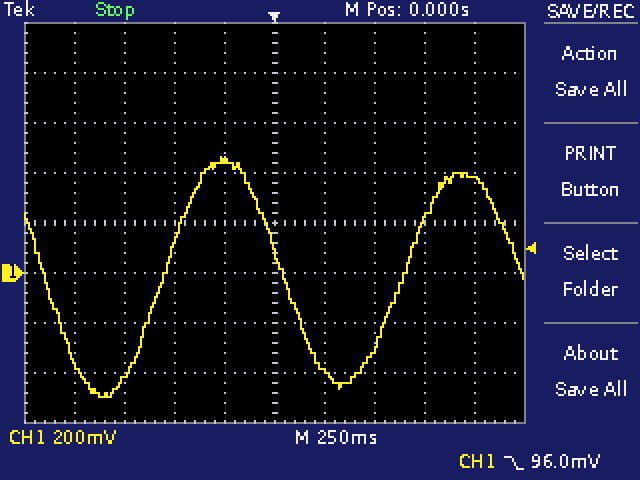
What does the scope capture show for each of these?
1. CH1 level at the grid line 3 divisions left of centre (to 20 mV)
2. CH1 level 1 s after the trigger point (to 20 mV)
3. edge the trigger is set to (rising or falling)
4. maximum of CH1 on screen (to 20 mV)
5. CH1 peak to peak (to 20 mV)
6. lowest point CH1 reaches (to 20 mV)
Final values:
-420 mV
380 mV
falling
460 mV
960 mV
-500 mV
